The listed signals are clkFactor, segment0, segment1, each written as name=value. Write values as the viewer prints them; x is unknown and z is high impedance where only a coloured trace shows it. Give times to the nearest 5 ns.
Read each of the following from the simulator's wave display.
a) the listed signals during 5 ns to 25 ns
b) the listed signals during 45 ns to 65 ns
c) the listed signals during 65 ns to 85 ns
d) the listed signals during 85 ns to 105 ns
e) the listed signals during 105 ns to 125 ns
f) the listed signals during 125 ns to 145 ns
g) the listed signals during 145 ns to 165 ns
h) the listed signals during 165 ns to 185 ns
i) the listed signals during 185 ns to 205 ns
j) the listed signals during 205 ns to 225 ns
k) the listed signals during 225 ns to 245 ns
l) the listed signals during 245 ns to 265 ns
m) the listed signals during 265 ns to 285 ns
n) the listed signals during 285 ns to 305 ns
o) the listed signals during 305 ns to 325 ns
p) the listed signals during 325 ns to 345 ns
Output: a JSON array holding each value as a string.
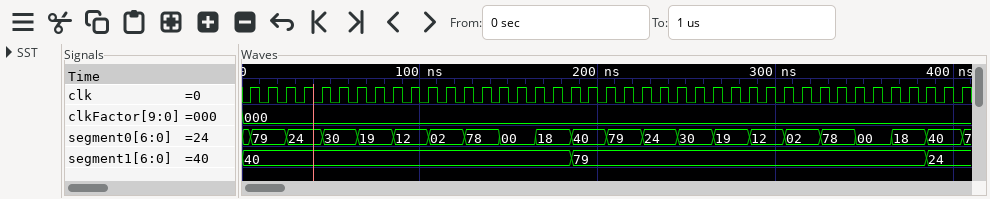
["clkFactor=000, segment0=79, segment1=40", "clkFactor=000, segment0=30, segment1=40", "clkFactor=000, segment0=19, segment1=40", "clkFactor=000, segment0=12, segment1=40", "clkFactor=000, segment0=02, segment1=40", "clkFactor=000, segment0=78, segment1=40", "clkFactor=000, segment0=00, segment1=40", "clkFactor=000, segment0=18, segment1=40", "clkFactor=000, segment0=40, segment1=79", "clkFactor=000, segment0=79, segment1=79", "clkFactor=000, segment0=24, segment1=79", "clkFactor=000, segment0=30, segment1=79", "clkFactor=000, segment0=19, segment1=79", "clkFactor=000, segment0=12, segment1=79", "clkFactor=000, segment0=02, segment1=79", "clkFactor=000, segment0=78, segment1=79"]
